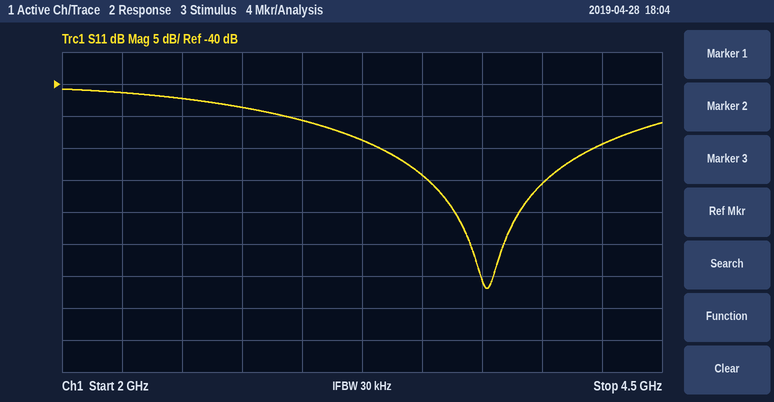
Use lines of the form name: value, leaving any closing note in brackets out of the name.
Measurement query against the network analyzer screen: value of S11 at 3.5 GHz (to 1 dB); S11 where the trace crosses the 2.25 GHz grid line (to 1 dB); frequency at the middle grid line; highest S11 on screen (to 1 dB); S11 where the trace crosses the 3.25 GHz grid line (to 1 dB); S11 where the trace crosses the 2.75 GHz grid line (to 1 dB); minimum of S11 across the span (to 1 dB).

value of S11 at 3.5 GHz: -54 dB
S11 where the trace crosses the 2.25 GHz grid line: -41 dB
frequency at the middle grid line: 3.25 GHz
highest S11 on screen: -41 dB
S11 where the trace crosses the 3.25 GHz grid line: -49 dB
S11 where the trace crosses the 2.75 GHz grid line: -44 dB
minimum of S11 across the span: -72 dB
